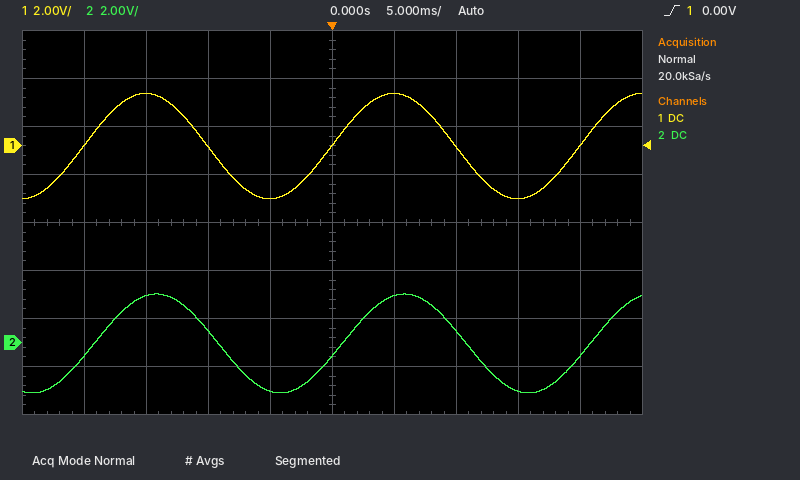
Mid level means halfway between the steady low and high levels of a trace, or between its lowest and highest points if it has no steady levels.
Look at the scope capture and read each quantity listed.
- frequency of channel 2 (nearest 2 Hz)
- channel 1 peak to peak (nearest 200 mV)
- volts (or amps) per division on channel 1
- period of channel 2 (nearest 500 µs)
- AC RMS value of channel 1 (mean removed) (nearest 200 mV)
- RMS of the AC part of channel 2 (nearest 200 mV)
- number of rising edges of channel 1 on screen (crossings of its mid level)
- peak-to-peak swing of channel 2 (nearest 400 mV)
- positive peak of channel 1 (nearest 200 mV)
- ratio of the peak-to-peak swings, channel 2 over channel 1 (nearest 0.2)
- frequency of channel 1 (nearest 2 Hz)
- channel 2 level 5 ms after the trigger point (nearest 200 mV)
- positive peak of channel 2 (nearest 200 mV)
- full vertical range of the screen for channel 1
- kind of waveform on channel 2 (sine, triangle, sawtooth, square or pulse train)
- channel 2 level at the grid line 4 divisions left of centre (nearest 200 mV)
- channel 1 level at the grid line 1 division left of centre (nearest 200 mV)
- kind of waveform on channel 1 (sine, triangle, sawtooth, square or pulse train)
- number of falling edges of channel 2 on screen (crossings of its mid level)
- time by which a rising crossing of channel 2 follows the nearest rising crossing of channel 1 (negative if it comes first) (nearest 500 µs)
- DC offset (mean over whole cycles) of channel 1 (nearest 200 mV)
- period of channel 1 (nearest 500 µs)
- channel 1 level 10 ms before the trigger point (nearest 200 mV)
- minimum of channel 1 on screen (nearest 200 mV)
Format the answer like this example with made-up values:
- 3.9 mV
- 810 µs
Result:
- 50 Hz
- 4.4 V
- 2 V
- 20.0 ms
- 1.6 V
- 1.4 V
- 3
- 4.0 V
- 2.2 V
- 1.0
- 50 Hz
- 2.0 V
- 2.0 V
- 16 V
- sine
- -600 mV
- -2.2 V
- sine
- 2
- +1.0 ms
- 0.0 V
- 20.0 ms
- 0.0 V
- -2.2 V
